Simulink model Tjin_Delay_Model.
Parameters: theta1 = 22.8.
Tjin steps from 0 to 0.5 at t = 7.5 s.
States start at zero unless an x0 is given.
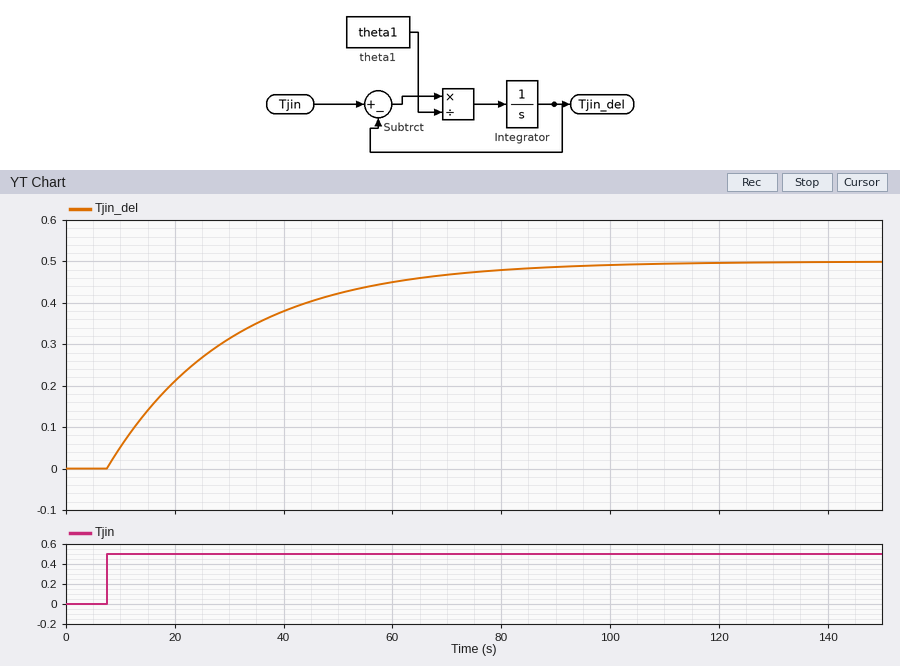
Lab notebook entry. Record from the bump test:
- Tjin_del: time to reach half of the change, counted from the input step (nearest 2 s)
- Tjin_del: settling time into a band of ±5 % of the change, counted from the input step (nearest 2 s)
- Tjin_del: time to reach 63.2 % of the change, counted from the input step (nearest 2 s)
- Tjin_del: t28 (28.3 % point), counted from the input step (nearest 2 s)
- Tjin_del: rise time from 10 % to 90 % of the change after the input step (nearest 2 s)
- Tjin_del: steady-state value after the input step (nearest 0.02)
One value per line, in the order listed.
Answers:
16 s
68 s
22 s
8 s
50 s
0.50
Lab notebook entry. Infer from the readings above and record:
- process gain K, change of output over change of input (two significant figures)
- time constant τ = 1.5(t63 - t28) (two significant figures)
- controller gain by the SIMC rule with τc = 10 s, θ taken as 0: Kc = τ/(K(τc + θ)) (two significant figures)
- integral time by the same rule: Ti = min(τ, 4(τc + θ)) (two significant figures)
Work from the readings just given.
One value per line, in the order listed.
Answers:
1.0
21 s
2.1
21 s
